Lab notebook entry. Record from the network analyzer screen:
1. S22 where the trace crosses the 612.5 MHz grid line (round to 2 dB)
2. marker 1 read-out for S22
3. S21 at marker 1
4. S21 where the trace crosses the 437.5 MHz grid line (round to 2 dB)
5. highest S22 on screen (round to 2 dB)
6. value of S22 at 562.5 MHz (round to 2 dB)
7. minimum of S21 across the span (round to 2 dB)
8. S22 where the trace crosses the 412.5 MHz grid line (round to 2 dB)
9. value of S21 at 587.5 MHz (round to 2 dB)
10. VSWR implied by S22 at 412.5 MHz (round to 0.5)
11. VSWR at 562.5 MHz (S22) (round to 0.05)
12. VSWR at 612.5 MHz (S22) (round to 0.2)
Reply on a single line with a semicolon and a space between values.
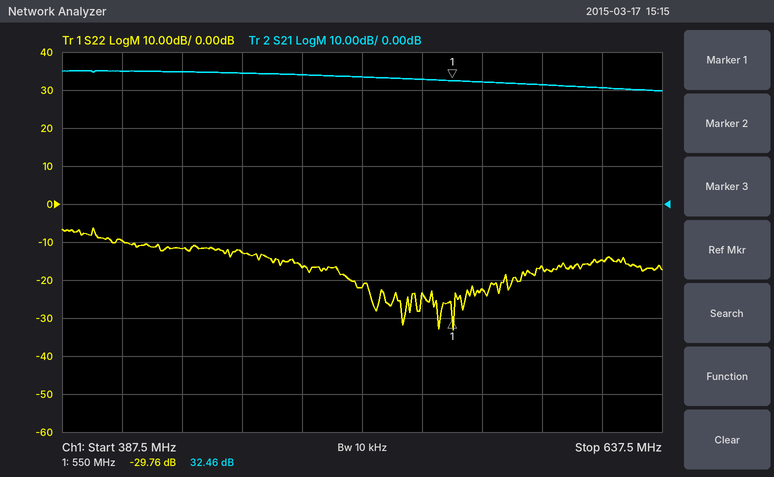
-14 dB; -29.76 dB; 32.46 dB; 34 dB; -6 dB; -22 dB; 30 dB; -10 dB; 32 dB; 2.0; 1.15; 1.4
